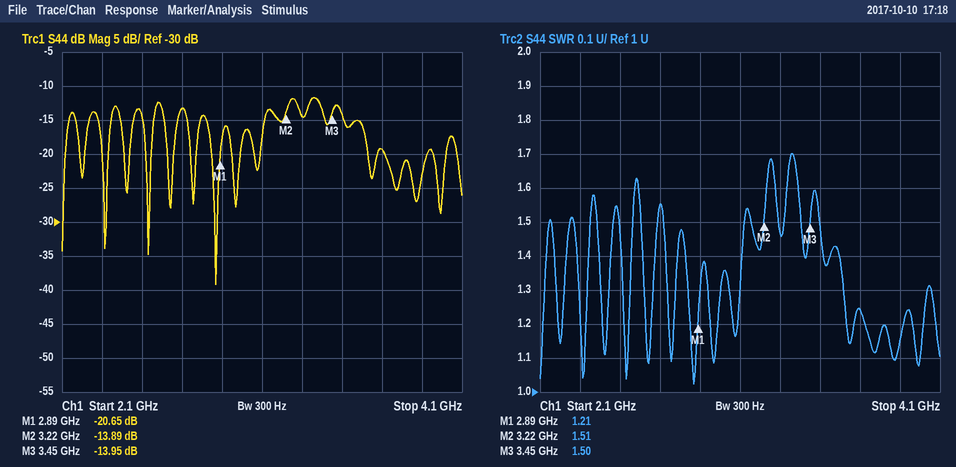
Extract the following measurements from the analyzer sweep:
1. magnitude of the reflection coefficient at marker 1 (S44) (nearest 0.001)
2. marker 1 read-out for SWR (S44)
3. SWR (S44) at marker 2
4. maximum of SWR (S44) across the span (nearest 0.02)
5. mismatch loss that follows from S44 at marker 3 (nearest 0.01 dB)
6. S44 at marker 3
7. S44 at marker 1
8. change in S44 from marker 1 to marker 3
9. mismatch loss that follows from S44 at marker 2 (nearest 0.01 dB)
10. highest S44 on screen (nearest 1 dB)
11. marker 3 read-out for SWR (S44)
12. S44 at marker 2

0.093
1.21
1.51
1.70
0.18 dB
-13.95 dB
-20.65 dB
6.70 dB
0.18 dB
-12 dB
1.50
-13.89 dB
